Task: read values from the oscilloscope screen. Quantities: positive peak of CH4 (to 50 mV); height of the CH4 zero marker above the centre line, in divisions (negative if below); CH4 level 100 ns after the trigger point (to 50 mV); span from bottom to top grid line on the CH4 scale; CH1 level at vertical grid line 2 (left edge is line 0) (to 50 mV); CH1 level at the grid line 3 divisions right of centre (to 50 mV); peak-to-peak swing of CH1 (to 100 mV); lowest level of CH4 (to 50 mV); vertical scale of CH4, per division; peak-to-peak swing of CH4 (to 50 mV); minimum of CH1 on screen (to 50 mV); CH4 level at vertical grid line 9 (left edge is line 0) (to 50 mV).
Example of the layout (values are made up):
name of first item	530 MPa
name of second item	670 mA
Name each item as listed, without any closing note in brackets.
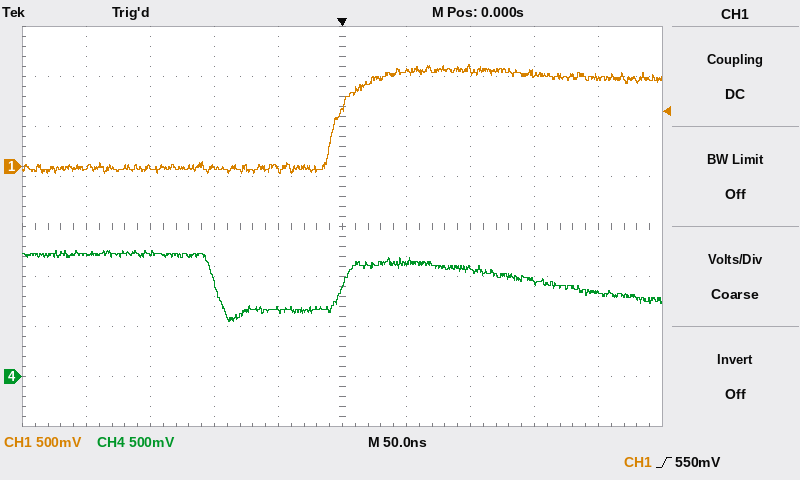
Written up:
positive peak of CH4	1.25 V
height of the CH4 zero marker above the centre line, in divisions	-3.0 div
CH4 level 100 ns after the trigger point	1.10 V
span from bottom to top grid line on the CH4 scale	4 V
CH1 level at vertical grid line 2 (left edge is line 0)	0 mV
CH1 level at the grid line 3 divisions right of centre	950 mV
peak-to-peak swing of CH1	1.10 V
lowest level of CH4	550 mV
vertical scale of CH4, per division	500 mV
peak-to-peak swing of CH4	700 mV
minimum of CH1 on screen	-50 mV
CH4 level at vertical grid line 9 (left edge is line 0)	850 mV
